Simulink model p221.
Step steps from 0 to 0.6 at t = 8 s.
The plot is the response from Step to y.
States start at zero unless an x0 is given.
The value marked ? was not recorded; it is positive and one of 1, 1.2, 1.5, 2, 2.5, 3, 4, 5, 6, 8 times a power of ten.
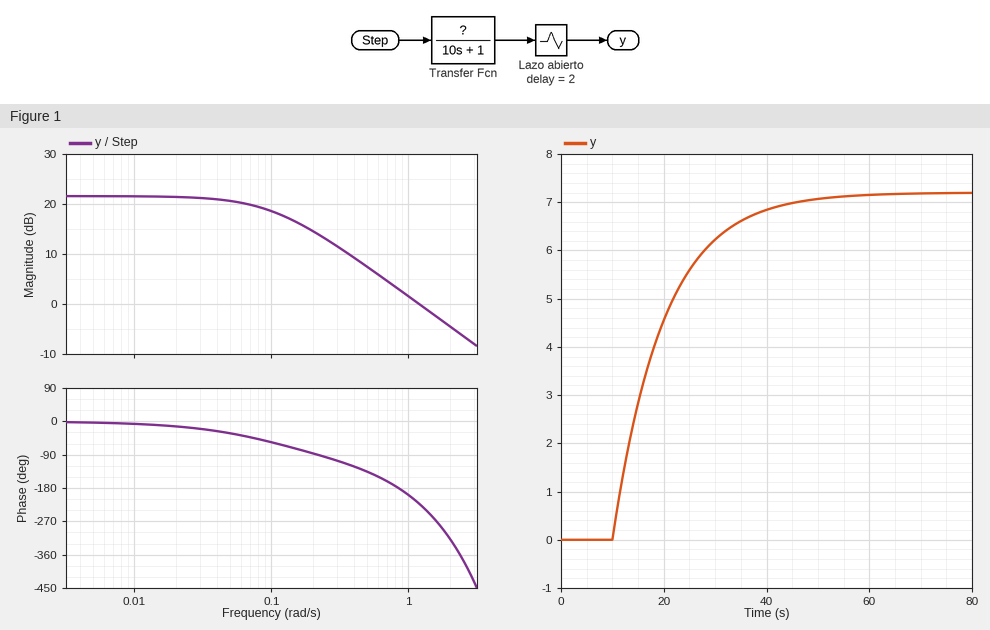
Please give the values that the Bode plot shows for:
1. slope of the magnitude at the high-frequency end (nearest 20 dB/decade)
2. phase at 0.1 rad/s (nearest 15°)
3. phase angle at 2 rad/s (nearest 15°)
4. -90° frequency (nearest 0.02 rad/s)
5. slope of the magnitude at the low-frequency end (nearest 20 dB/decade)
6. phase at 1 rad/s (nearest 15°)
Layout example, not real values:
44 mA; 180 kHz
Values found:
-20 dB/decade; -60°; -315°; 0.22 rad/s; 0 dB/decade; -195°
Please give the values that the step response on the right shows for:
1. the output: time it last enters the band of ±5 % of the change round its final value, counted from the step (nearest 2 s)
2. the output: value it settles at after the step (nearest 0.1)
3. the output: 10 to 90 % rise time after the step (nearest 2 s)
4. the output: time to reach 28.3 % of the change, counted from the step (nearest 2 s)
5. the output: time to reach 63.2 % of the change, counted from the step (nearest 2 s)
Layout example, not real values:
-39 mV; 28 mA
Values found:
32 s; 7.2; 22 s; 6 s; 12 s
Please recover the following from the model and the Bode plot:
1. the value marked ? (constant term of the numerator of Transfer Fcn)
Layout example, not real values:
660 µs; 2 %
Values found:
12
